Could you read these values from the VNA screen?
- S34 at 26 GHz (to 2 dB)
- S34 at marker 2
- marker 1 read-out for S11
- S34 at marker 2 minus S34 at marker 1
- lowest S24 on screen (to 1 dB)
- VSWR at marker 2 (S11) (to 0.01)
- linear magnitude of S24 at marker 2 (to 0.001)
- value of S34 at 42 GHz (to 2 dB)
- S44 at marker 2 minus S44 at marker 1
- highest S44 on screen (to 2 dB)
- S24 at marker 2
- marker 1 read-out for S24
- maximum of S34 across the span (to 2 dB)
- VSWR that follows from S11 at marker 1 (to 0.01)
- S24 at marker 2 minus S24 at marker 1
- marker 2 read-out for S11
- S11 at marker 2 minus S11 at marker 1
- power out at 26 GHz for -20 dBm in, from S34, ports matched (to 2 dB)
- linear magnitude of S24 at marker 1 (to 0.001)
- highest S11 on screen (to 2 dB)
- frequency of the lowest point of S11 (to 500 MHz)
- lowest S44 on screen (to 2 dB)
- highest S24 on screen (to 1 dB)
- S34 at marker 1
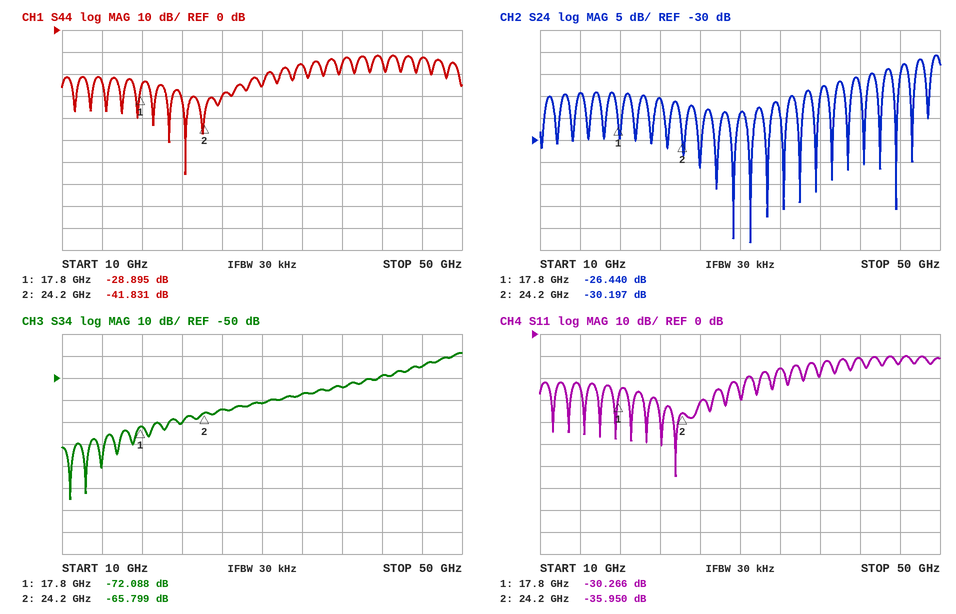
-64 dB
-65.799 dB
-30.266 dB
6.289 dB
-53 dB
1.03
0.031
-48 dB
-12.936 dB
-12 dB
-30.197 dB
-26.440 dB
-38 dB
1.06
-3.757 dB
-35.950 dB
-5.684 dB
-84 dBm
0.048
-10 dB
23.5 GHz
-66 dB
-11 dB
-72.088 dB
